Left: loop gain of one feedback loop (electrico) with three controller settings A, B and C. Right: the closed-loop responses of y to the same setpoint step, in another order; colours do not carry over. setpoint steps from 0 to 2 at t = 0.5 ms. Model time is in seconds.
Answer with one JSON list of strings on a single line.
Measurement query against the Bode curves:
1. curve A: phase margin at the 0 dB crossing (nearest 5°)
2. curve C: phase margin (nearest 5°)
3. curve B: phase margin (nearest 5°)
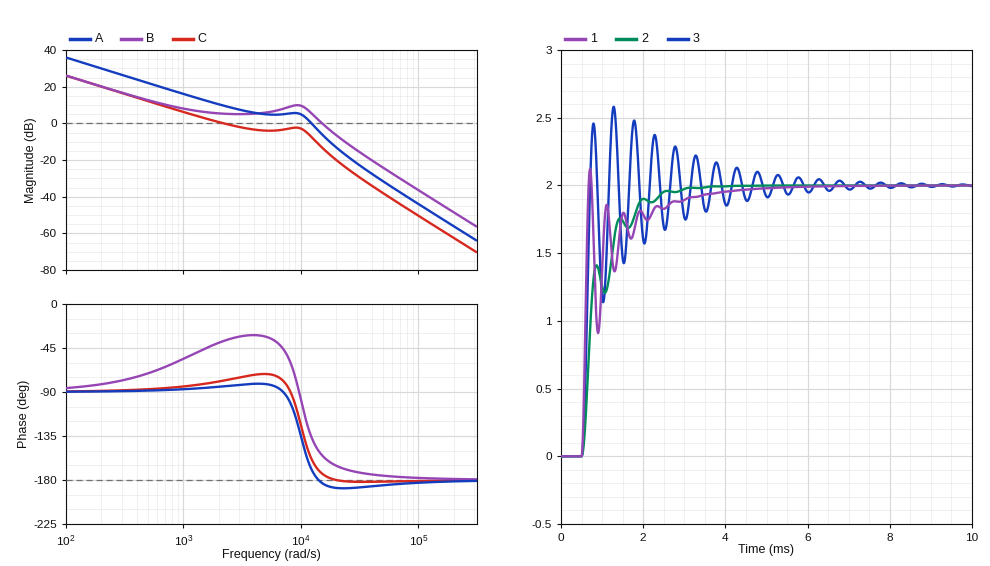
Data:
["10°", "100°", "25°"]
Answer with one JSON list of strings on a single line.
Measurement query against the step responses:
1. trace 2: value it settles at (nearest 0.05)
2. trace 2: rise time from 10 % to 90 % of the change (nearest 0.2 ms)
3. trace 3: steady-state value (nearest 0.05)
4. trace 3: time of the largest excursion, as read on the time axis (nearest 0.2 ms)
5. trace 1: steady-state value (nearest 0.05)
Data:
["2.00", "1.2 ms", "2.00", "1.2 ms", "2.00"]
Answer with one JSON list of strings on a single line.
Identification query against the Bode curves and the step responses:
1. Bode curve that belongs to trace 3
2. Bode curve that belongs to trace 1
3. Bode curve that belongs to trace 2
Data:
["A", "B", "C"]
